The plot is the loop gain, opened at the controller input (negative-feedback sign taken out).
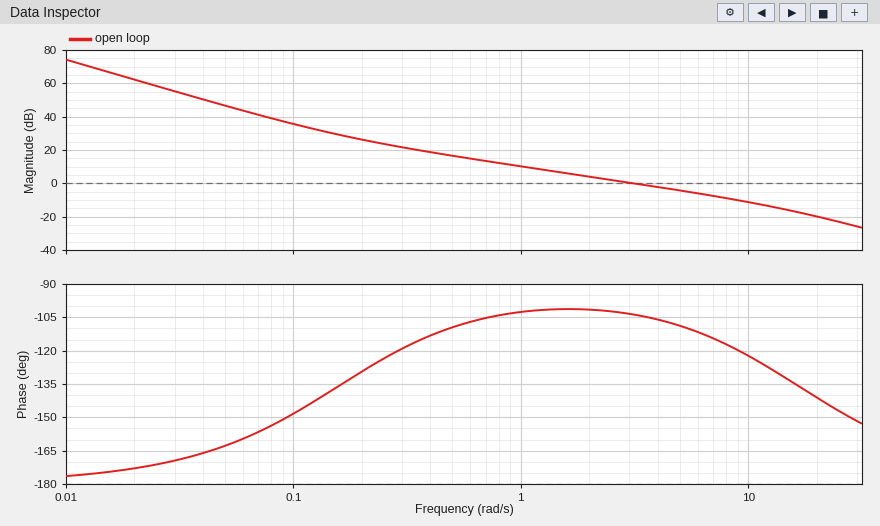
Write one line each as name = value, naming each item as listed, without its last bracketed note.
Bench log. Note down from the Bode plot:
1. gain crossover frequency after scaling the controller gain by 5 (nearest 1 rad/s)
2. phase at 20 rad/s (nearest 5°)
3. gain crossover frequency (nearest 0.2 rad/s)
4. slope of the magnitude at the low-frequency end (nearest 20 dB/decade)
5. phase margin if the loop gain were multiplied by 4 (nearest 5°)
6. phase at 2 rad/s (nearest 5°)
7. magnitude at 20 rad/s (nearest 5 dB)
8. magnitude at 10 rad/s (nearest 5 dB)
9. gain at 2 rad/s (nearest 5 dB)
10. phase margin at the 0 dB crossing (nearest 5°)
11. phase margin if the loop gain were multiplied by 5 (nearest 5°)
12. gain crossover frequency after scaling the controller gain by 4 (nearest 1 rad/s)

gain crossover frequency after scaling the controller gain by 5 = 13 rad/s
phase at 20 rad/s = -140°
gain crossover frequency = 3.2 rad/s
slope of the magnitude at the low-frequency end = -40 dB/decade
phase margin if the loop gain were multiplied by 4 = 55°
phase at 2 rad/s = -100°
magnitude at 20 rad/s = -20 dB
magnitude at 10 rad/s = -10 dB
gain at 2 rad/s = 5 dB
phase margin at the 0 dB crossing = 75°
phase margin if the loop gain were multiplied by 5 = 50°
gain crossover frequency after scaling the controller gain by 4 = 11 rad/s
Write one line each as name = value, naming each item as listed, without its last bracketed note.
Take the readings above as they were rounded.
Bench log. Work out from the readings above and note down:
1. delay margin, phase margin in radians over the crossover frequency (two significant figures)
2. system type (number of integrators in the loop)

delay margin, phase margin in radians over the crossover frequency = 0.41 s
system type = 2
